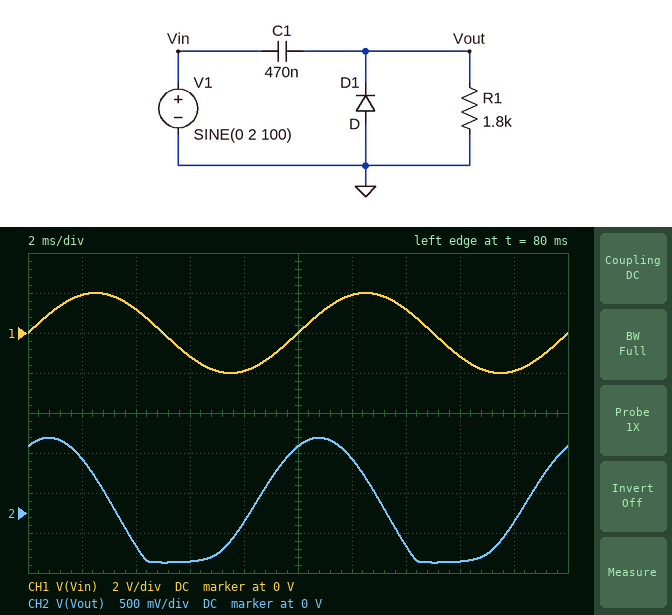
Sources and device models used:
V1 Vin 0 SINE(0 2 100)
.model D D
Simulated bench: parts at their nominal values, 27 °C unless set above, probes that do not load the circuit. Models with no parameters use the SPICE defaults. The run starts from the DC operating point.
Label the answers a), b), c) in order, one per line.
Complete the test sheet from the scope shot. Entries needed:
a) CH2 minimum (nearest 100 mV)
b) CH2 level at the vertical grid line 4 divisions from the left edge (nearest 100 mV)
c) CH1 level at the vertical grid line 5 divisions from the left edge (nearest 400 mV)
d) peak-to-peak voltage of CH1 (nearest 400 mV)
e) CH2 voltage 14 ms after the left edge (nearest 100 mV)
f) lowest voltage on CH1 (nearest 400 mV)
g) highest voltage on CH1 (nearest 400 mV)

a) -600 mV
b) -100 mV
c) 0 V
d) 4.0 V
e) -400 mV
f) -2.0 V
g) 2.0 V
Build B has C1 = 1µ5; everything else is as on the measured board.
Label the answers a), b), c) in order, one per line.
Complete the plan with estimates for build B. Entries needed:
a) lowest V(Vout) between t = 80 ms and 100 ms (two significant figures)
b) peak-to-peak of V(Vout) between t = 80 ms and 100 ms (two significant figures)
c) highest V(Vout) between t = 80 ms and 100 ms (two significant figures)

a) -670 mV
b) 2.6 V
c) 1.9 V
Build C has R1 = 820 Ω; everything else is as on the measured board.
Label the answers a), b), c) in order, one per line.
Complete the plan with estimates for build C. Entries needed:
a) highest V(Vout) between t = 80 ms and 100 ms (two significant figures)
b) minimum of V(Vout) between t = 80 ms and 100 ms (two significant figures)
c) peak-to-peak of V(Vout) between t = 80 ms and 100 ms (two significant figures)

a) 470 mV
b) -470 mV
c) 940 mV
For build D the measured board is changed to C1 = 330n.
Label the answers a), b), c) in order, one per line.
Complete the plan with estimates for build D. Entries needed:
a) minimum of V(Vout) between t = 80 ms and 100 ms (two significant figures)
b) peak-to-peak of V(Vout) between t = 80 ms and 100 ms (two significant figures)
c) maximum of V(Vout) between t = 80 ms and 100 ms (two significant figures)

a) -590 mV
b) 1.3 V
c) 700 mV
